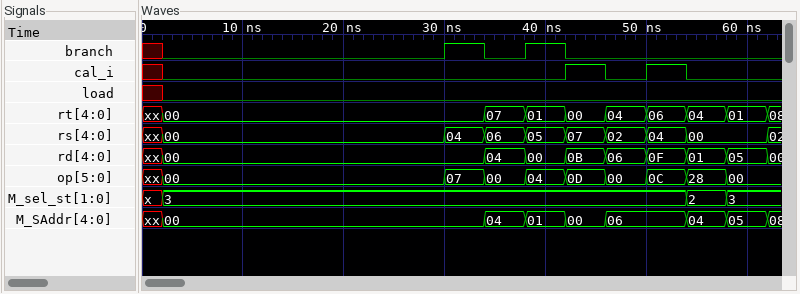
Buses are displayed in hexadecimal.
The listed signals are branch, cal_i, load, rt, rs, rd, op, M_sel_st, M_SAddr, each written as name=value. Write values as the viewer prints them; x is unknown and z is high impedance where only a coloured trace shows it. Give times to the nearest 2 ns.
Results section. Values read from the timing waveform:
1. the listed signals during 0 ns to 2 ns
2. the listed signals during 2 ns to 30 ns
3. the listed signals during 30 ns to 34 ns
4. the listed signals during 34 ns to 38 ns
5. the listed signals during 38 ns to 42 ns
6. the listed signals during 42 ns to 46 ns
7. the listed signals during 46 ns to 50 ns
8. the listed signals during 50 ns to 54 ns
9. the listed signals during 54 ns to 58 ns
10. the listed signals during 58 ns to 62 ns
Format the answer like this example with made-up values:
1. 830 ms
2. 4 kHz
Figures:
1. branch=x, cal_i=x, load=x, rt=xx, rs=xx, rd=xx, op=xx, M_sel_st=x, M_SAddr=xx
2. branch=0, cal_i=0, load=0, rt=00, rs=00, rd=00, op=00, M_sel_st=3, M_SAddr=00
3. branch=1, cal_i=0, load=0, rt=00, rs=04, rd=00, op=07, M_sel_st=3, M_SAddr=00
4. branch=0, cal_i=0, load=0, rt=07, rs=06, rd=04, op=00, M_sel_st=3, M_SAddr=04
5. branch=1, cal_i=0, load=0, rt=01, rs=05, rd=00, op=04, M_sel_st=3, M_SAddr=01
6. branch=0, cal_i=1, load=0, rt=00, rs=07, rd=0B, op=0D, M_sel_st=3, M_SAddr=00
7. branch=0, cal_i=0, load=0, rt=04, rs=02, rd=06, op=00, M_sel_st=3, M_SAddr=06
8. branch=0, cal_i=1, load=0, rt=06, rs=04, rd=0F, op=0C, M_sel_st=3, M_SAddr=06
9. branch=0, cal_i=0, load=0, rt=04, rs=00, rd=01, op=28, M_sel_st=2, M_SAddr=04
10. branch=0, cal_i=0, load=0, rt=01, rs=00, rd=05, op=00, M_sel_st=3, M_SAddr=05
